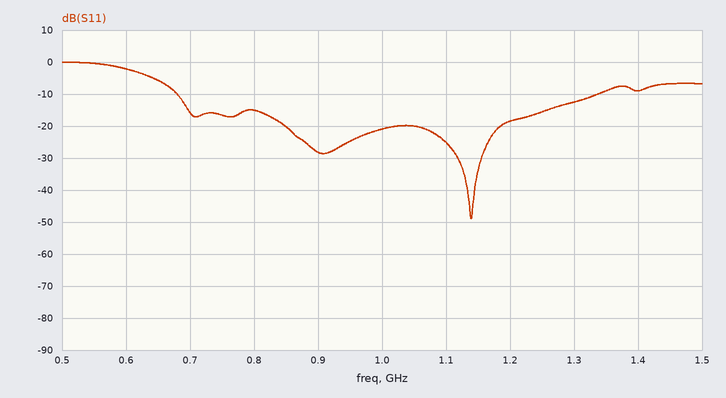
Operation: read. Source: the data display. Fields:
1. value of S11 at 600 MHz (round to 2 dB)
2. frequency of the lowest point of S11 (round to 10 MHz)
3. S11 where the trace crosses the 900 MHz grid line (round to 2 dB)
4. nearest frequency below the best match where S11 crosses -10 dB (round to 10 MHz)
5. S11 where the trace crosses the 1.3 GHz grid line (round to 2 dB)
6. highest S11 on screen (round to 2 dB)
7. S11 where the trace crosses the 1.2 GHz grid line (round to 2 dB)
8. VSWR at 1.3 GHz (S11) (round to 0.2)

-2 dB
1.14 GHz
-28 dB
680 MHz
-12 dB
0 dB
-18 dB
1.6
